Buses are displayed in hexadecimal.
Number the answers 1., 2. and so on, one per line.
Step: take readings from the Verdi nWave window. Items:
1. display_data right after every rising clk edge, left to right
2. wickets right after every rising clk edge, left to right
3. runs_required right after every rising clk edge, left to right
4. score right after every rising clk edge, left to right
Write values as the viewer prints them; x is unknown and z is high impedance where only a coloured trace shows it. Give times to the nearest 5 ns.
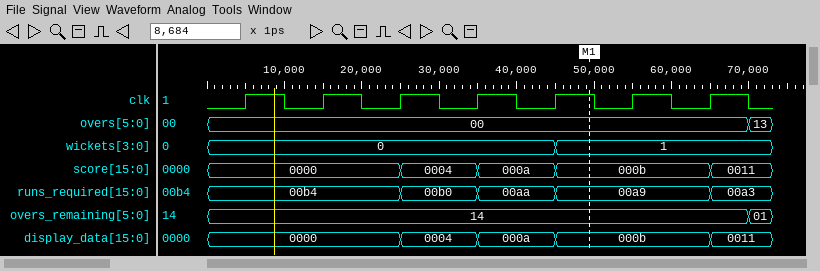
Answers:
1. 0000, 0000, 0004, 000a, 000b, 000b, 0011
2. 0, 0, 0, 0, 1, 1, 1
3. 00b4, 00b4, 00b0, 00aa, 00a9, 00a9, 00a3
4. 0000, 0000, 0004, 000a, 000b, 000b, 0011
